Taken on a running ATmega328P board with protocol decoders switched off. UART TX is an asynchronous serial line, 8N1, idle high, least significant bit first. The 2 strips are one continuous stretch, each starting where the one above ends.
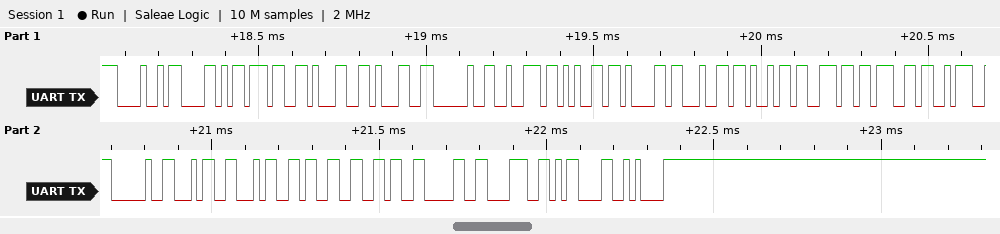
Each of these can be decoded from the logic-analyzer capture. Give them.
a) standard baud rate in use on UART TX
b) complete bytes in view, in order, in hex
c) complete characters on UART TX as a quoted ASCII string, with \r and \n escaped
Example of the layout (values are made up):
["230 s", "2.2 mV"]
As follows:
["57600 baud", "48 58 37 31 31 20 72 65 61 64 69 6E 67 3A 20 34 34 33 36 30 38 0D 0A", "\"HX711 reading: 443608\\r\\n\""]
